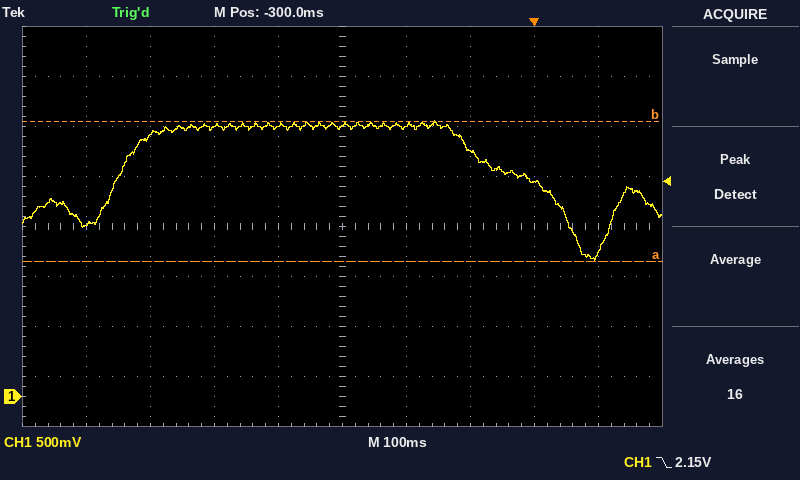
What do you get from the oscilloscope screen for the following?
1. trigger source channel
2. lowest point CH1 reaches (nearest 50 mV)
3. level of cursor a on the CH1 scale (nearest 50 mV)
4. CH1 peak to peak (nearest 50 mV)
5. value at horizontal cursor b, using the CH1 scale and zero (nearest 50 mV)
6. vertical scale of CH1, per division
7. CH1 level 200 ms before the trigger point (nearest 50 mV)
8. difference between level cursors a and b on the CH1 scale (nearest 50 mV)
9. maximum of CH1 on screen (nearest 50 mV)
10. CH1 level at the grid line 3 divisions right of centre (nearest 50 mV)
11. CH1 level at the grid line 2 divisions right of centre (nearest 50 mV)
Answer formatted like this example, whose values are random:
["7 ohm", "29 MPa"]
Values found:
["CH1", "1.35 V", "1.35 V", "1.40 V", "2.75 V", "500 mV", "2.70 V", "1.40 V", "2.75 V", "2.15 V", "2.45 V"]
